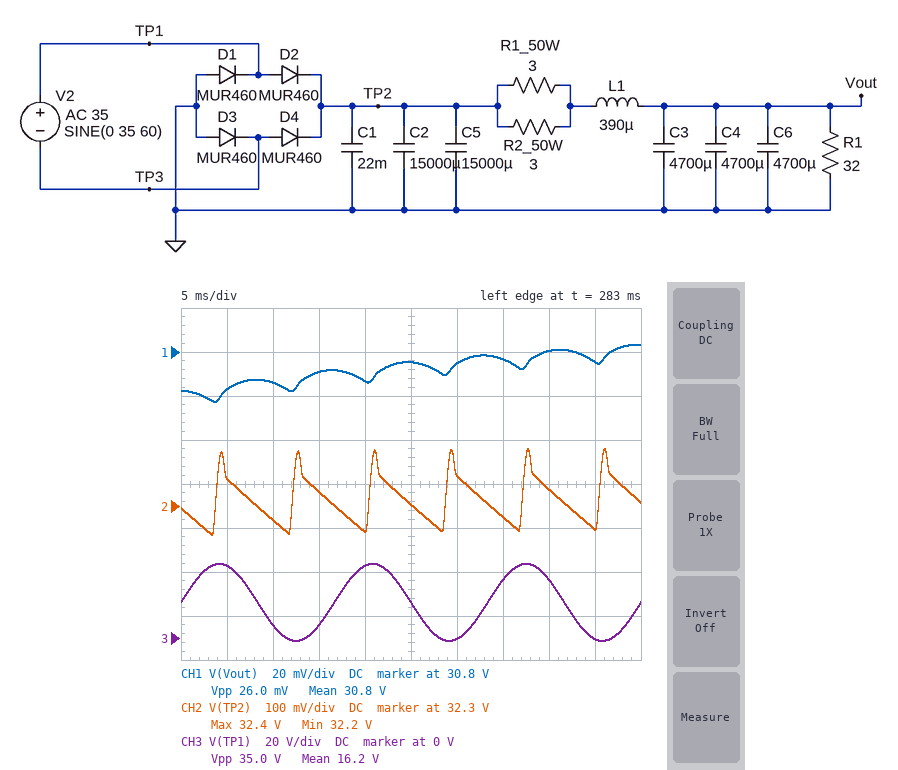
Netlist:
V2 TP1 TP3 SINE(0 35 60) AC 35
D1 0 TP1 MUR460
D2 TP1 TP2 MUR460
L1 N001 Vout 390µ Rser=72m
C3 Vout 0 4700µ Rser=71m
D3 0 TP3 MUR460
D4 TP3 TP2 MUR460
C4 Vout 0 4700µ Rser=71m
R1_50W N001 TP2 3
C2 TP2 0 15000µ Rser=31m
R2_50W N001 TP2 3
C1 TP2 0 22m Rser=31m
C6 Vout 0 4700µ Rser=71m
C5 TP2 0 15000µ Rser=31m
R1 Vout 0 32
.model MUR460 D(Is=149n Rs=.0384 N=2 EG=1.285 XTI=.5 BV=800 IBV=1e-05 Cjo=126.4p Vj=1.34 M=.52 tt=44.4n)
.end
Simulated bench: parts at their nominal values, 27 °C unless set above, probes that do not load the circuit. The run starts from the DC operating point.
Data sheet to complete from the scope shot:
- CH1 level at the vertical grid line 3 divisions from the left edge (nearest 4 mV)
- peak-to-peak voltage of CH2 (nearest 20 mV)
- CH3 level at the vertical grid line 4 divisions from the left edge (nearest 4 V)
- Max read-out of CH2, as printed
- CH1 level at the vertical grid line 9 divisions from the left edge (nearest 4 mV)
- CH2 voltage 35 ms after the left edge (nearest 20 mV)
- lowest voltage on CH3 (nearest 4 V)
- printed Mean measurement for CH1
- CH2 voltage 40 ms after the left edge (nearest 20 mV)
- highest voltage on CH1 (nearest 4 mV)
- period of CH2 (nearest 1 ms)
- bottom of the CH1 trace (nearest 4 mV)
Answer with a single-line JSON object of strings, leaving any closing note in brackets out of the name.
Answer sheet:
{"CH1 level at the vertical grid line 3 divisions from the left edge": "30.792 V", "peak-to-peak voltage of CH2": "200 mV", "CH3 level at the vertical grid line 4 divisions from the left edge": "32 V", "Max read-out of CH2, as printed": "32.4 V", "CH1 level at the vertical grid line 9 divisions from the left edge": "30.796 V", "CH2 voltage 35 ms after the left edge": "32.28 V", "lowest voltage on CH3": "0 V", "printed Mean measurement for CH1": "30.8 V", "CH2 voltage 40 ms after the left edge": "32.34 V", "highest voltage on CH1": "30.804 V", "period of CH2": "8 ms", "bottom of the CH1 trace": "30.776 V"}
